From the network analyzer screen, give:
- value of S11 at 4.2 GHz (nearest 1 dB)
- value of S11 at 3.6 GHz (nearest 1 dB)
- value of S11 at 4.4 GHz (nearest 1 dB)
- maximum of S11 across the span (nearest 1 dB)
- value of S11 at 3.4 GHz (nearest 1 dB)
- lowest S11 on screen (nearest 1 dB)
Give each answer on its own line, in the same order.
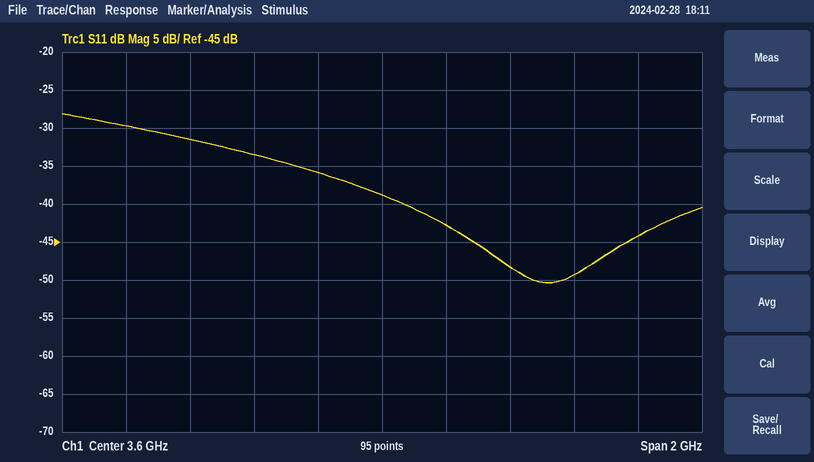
-49 dB
-39 dB
-44 dB
-28 dB
-36 dB
-50 dB
